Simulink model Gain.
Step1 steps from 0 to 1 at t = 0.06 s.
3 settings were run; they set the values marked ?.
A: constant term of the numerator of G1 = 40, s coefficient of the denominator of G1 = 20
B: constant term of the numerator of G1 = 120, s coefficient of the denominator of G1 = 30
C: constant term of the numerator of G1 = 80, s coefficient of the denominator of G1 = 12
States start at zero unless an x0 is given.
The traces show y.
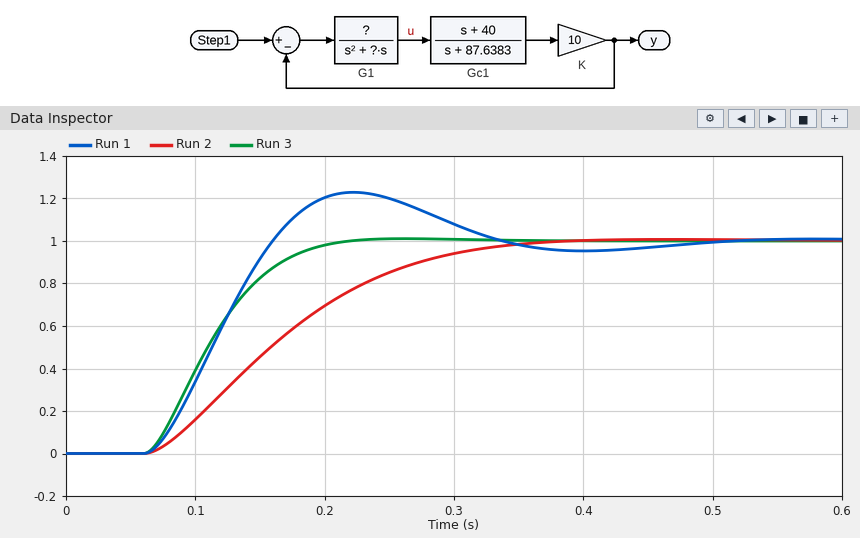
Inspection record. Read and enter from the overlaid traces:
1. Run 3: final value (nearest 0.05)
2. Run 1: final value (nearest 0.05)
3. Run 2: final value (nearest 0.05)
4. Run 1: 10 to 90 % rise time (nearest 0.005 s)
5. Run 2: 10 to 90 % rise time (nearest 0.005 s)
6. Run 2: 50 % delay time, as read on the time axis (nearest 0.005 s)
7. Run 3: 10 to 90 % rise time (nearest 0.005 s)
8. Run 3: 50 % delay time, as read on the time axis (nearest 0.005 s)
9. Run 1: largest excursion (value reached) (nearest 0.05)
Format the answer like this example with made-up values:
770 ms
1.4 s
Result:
1.00
1.00
1.00
0.070 s
0.185 s
0.160 s
0.090 s
0.110 s
1.25
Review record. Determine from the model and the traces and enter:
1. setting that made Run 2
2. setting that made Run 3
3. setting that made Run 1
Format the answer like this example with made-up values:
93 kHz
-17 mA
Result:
A
B
C
